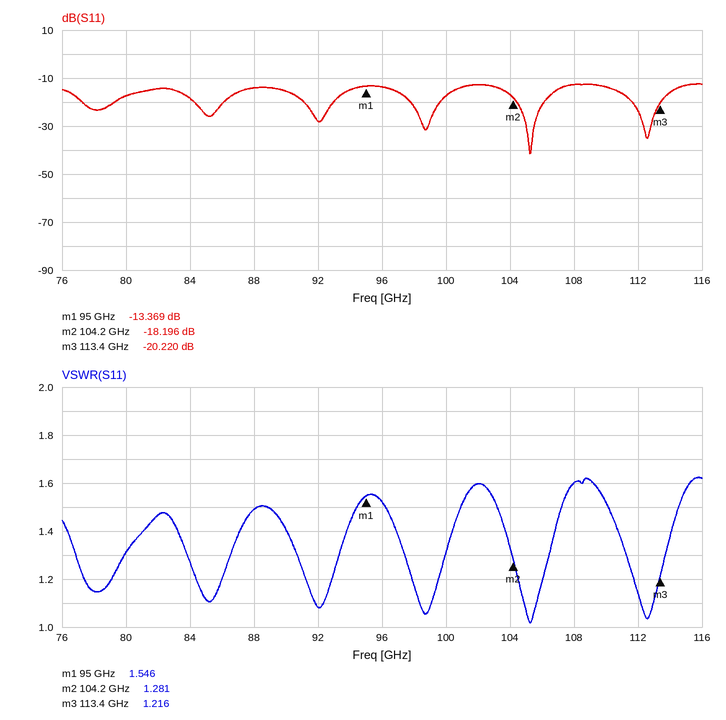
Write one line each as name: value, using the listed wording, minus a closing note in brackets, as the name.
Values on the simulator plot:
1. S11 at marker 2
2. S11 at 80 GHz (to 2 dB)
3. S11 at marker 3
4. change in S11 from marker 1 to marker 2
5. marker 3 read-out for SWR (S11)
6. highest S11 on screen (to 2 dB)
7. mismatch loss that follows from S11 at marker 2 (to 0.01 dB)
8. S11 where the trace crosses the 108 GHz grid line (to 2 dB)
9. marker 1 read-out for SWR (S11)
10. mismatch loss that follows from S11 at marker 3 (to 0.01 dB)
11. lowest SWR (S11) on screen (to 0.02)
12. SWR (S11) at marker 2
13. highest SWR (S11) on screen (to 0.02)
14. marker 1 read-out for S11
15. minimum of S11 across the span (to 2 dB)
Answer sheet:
S11 at marker 2: -18.196 dB
S11 at 80 GHz: -18 dB
S11 at marker 3: -20.220 dB
change in S11 from marker 1 to marker 2: -4.827 dB
marker 3 read-out for SWR: 1.216
highest S11 on screen: -12 dB
mismatch loss that follows from S11 at marker 2: 0.07 dB
S11 where the trace crosses the 108 GHz grid line: -12 dB
marker 1 read-out for SWR: 1.546
mismatch loss that follows from S11 at marker 3: 0.04 dB
lowest SWR (S11) on screen: 1.02
SWR (S11) at marker 2: 1.281
highest SWR (S11) on screen: 1.62
marker 1 read-out for S11: -13.369 dB
minimum of S11 across the span: -42 dB
